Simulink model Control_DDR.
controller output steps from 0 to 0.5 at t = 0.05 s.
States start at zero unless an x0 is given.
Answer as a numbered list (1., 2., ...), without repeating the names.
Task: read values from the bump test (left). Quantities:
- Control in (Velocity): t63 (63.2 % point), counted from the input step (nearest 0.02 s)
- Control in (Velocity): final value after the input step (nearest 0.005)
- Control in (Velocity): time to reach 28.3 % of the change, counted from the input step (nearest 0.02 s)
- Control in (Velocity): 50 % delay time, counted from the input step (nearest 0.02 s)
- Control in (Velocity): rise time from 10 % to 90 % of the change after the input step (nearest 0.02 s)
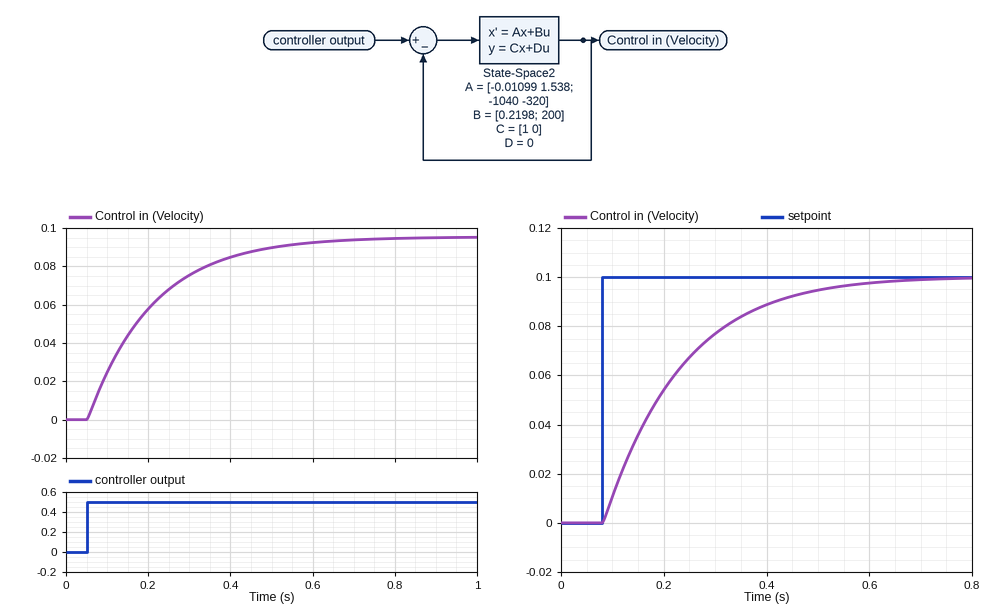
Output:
1. 0.16 s
2. 0.095
3. 0.06 s
4. 0.12 s
5. 0.34 s
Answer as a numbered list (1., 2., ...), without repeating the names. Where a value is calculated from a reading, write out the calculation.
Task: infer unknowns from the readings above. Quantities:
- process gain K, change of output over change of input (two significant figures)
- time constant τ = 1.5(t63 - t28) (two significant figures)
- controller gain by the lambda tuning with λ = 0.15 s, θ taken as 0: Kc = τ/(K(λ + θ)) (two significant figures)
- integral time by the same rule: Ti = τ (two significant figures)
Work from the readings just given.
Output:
1. (0.095 - 0) / 0.5 = 0.19
2. 1.5 × (0.16 - 0.06) = 0.15 s
3. 0.15 / (0.19 × (0.15 + 0)) = 5.3
4. 0.15 s
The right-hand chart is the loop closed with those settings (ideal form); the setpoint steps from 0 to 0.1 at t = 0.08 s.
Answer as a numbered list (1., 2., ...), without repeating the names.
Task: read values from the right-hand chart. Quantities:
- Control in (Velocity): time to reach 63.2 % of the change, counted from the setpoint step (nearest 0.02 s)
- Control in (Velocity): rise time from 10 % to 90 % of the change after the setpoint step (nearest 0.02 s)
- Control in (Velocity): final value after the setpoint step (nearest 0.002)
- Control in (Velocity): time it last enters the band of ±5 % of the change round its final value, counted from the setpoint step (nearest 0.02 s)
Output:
1. 0.16 s
2. 0.32 s
3. 0.100
4. 0.42 s
